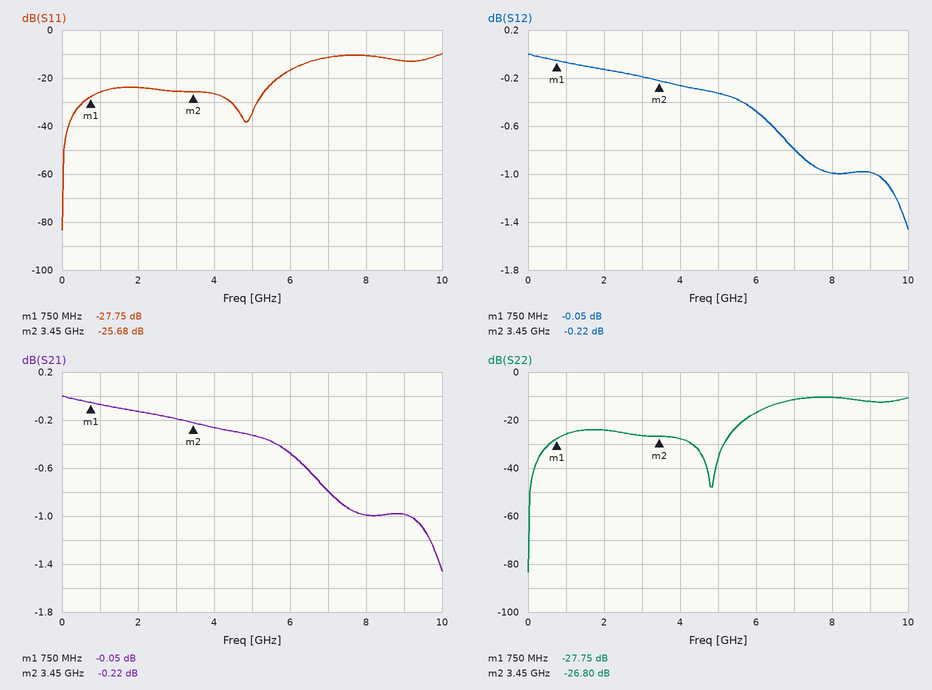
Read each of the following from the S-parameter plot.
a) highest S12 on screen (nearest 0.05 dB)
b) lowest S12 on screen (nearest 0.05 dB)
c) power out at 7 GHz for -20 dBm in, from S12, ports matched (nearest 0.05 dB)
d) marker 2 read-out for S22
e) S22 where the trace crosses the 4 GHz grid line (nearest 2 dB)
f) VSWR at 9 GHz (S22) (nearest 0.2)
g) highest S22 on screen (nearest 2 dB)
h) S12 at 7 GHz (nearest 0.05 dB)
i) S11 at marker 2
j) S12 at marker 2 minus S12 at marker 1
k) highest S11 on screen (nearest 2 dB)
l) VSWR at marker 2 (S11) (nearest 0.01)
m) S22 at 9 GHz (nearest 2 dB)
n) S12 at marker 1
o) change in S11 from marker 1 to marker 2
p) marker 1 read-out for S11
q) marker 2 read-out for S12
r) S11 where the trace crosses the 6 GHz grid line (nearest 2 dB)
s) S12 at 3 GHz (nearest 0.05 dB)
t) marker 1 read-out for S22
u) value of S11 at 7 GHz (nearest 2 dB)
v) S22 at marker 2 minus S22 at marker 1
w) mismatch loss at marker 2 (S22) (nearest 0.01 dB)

0.00 dB
-1.45 dB
-20.80 dBm
-26.80 dB
-28 dB
1.6
-10 dB
-0.80 dB
-25.68 dB
-0.17 dB
-10 dB
1.11
-12 dB
-0.05 dB
2.07 dB
-27.75 dB
-0.22 dB
-16 dB
-0.20 dB
-27.75 dB
-12 dB
0.95 dB
0.01 dB
